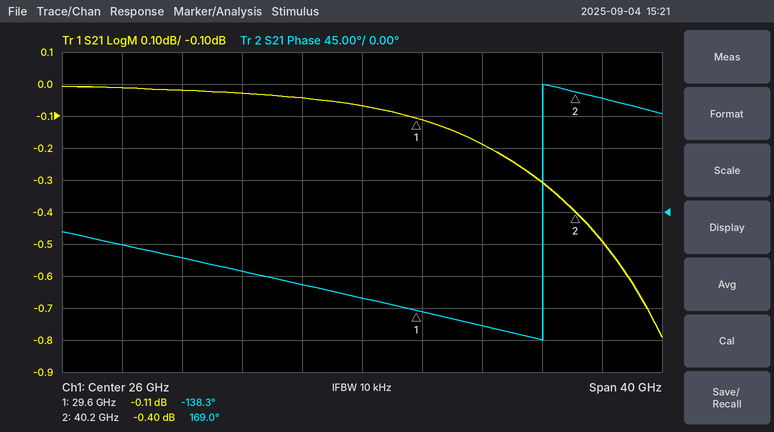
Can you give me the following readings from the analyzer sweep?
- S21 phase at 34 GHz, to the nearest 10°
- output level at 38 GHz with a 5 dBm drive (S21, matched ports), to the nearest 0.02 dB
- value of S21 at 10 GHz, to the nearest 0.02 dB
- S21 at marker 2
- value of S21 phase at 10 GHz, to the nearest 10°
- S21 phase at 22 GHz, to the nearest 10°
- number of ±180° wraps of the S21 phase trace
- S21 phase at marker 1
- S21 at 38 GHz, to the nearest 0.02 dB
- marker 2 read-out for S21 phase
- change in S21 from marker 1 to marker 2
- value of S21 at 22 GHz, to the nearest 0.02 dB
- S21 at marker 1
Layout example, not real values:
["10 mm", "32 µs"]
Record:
["-160°", "4.70 dBm", "-0.02 dB", "-0.40 dB", "-50°", "-100°", "1", "-138.3°", "-0.30 dB", "169.0°", "-0.29 dB", "-0.04 dB", "-0.11 dB"]
